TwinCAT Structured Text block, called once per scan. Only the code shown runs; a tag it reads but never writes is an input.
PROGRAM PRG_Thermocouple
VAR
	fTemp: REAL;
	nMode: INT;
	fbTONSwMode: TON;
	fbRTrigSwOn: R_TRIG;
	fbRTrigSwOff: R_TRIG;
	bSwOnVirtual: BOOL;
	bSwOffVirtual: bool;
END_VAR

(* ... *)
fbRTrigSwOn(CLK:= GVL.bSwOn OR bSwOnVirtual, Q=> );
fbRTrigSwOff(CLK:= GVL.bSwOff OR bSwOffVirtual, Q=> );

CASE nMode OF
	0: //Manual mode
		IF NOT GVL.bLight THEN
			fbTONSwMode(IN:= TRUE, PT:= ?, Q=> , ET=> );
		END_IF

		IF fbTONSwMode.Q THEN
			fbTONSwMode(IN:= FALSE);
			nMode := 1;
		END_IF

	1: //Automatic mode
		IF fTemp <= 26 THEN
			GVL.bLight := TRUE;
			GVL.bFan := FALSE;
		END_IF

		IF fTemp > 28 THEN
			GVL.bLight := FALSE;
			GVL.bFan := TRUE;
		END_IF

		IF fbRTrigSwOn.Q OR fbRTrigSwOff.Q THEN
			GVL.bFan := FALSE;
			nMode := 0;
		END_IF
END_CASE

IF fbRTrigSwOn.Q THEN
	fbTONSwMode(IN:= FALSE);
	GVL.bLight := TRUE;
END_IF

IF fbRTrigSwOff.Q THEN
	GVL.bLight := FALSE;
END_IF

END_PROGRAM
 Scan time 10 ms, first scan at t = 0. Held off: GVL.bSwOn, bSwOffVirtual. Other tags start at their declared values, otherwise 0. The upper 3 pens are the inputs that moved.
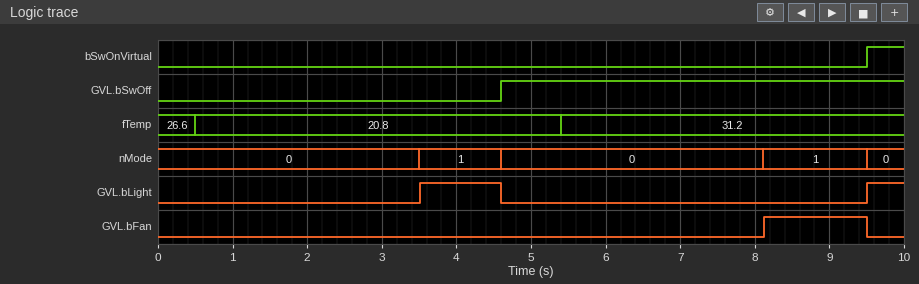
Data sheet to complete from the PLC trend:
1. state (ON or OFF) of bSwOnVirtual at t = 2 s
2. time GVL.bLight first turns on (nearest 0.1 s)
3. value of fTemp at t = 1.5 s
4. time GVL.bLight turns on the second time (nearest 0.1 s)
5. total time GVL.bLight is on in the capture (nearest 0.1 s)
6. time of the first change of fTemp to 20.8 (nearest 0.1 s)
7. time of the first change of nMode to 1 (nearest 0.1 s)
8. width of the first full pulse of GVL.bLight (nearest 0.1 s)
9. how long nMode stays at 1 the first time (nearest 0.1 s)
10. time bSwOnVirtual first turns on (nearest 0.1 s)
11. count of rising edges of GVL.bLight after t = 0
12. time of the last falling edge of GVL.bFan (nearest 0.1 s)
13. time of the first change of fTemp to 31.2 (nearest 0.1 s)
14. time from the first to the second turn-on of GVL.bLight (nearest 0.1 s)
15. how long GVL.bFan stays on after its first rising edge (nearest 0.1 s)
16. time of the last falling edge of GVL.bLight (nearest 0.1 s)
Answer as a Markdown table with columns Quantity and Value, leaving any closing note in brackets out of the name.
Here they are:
| Quantity | Value |
|---|---|
| state (ON or OFF) of bSwOnVirtual at t = 2 s | OFF |
| time GVL.bLight first turns on | 3.5 s |
| value of fTemp at t = 1.5 s | 20.8 |
| time GVL.bLight turns on the second time | 9.5 s |
| total time GVL.bLight is on in the capture | 1.6 s |
| time of the first change of fTemp to 20.8 | 0.5 s |
| time of the first change of nMode to 1 | 3.5 s |
| width of the first full pulse of GVL.bLight | 1.1 s |
| how long nMode stays at 1 the first time | 1.1 s |
| time bSwOnVirtual first turns on | 9.5 s |
| count of rising edges of GVL.bLight after t = 0 | 2 |
| time of the last falling edge of GVL.bFan | 9.5 s |
| time of the first change of fTemp to 31.2 | 5.4 s |
| time from the first to the second turn-on of GVL.bLight | 6.0 s |
| how long GVL.bFan stays on after its first rising edge | 1.4 s |
| time of the last falling edge of GVL.bLight | 4.6 s |
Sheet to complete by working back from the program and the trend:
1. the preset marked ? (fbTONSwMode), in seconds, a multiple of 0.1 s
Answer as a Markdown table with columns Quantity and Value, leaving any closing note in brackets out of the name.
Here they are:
| Quantity | Value |
|---|---|
| the preset marked ? (fbTONSwMode), in seconds, a multiple of 0.1 s | 3.5 s |
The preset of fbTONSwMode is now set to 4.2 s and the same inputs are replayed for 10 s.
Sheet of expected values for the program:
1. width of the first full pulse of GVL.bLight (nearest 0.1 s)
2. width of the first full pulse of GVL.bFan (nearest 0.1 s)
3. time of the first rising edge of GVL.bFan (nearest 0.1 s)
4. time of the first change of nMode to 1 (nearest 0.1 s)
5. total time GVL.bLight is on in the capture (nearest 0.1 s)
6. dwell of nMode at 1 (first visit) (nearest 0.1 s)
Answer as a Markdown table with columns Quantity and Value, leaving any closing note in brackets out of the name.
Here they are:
| Quantity | Value |
|---|---|
| width of the first full pulse of GVL.bLight | 0.4 s |
| width of the first full pulse of GVL.bFan | 0.7 s |
| time of the first rising edge of GVL.bFan | 8.8 s |
| time of the first change of nMode to 1 | 4.2 s |
| total time GVL.bLight is on in the capture | 0.9 s |
| dwell of nMode at 1 (first visit) | 0.4 s |
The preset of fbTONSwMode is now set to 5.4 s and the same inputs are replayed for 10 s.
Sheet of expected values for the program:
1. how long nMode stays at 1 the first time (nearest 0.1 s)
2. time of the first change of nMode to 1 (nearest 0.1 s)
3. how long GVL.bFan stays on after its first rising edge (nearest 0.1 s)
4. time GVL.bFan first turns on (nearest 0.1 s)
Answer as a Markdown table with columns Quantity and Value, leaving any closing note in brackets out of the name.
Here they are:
| Quantity | Value |
|---|---|
| how long nMode stays at 1 the first time | 4.1 s |
| time of the first change of nMode to 1 | 5.4 s |
| how long GVL.bFan stays on after its first rising edge | 4.1 s |
| time GVL.bFan first turns on | 5.4 s |
